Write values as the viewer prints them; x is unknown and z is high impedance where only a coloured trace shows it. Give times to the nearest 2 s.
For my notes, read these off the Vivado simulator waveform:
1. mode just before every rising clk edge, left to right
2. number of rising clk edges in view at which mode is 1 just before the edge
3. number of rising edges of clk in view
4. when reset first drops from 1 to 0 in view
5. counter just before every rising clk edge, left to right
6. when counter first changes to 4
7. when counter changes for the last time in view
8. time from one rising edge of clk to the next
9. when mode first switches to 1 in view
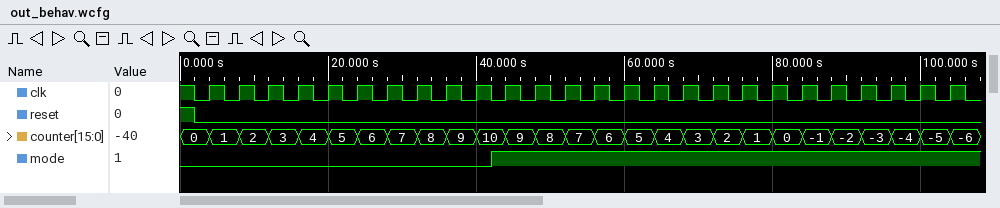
0 0 0 0 0 0 0 0 0 0 1 1 1 1 1 1 1 1 1 1 1 1 1 1 1 1
16
26
2 s
0, 1, 2, 3, 4, 5, 6, 7, 8, 9, 10, 9, 8, 7, 6, 5, 4, 3, 2, 1, 0, -1, -2, -3, -4, -5
16 s
104 s
4 s
42 s
